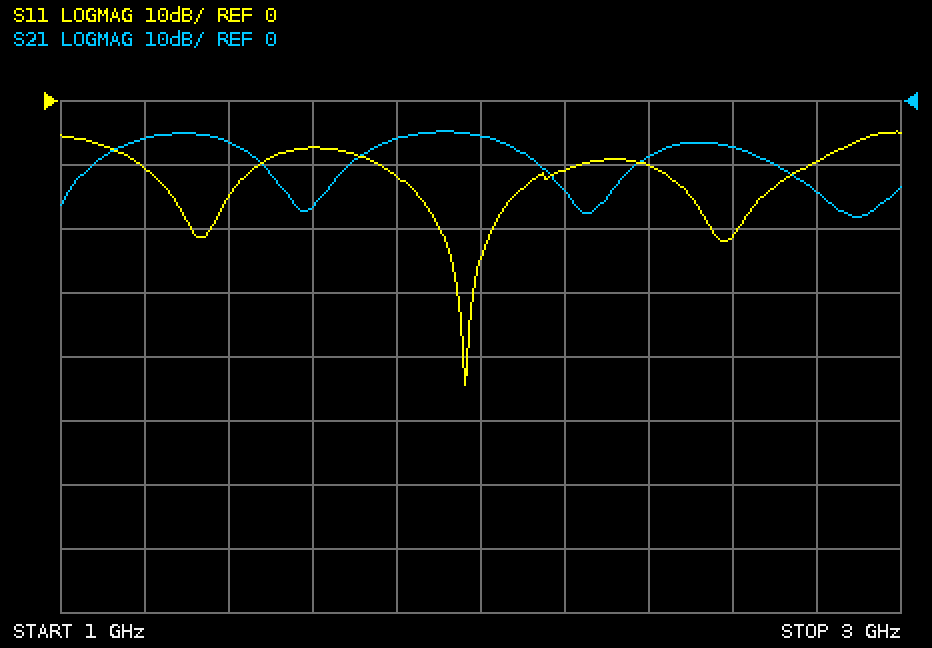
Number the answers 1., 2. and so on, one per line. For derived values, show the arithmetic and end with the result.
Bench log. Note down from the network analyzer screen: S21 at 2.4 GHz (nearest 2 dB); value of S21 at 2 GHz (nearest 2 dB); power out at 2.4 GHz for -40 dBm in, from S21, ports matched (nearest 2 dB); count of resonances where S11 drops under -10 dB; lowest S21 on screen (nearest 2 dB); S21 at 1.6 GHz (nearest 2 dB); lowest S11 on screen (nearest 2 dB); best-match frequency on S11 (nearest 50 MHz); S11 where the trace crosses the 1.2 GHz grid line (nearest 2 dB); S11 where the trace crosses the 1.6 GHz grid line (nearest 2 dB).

1. -8 dB
2. -6 dB
3. -40 dBm + (-8 dB) = -48 dBm
4. 3
5. -18 dB
6. -16 dB
7. -44 dB
8. 1.95 GHz
9. -10 dB
10. -8 dB
